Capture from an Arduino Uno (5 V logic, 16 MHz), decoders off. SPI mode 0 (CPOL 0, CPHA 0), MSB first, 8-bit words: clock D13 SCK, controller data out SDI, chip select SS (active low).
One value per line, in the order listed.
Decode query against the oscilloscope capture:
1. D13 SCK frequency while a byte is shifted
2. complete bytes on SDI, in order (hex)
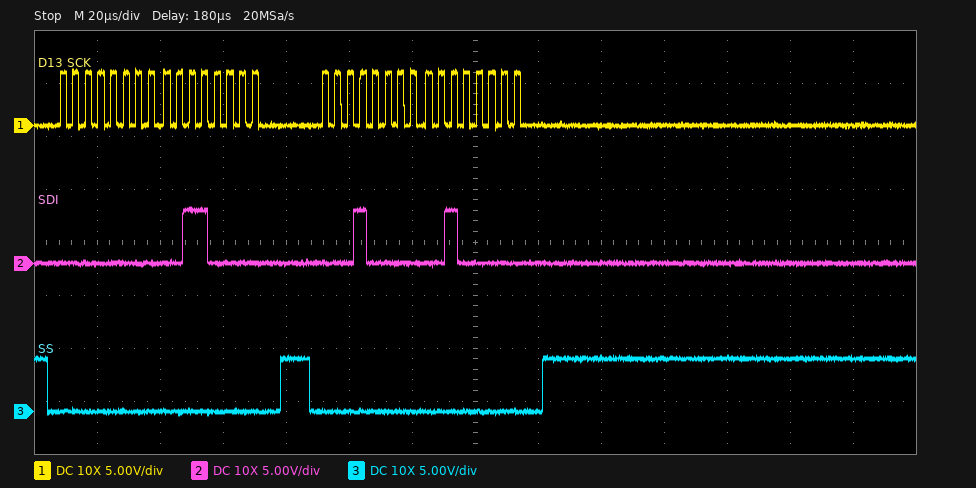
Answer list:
250 kHz
00 30 10 20
